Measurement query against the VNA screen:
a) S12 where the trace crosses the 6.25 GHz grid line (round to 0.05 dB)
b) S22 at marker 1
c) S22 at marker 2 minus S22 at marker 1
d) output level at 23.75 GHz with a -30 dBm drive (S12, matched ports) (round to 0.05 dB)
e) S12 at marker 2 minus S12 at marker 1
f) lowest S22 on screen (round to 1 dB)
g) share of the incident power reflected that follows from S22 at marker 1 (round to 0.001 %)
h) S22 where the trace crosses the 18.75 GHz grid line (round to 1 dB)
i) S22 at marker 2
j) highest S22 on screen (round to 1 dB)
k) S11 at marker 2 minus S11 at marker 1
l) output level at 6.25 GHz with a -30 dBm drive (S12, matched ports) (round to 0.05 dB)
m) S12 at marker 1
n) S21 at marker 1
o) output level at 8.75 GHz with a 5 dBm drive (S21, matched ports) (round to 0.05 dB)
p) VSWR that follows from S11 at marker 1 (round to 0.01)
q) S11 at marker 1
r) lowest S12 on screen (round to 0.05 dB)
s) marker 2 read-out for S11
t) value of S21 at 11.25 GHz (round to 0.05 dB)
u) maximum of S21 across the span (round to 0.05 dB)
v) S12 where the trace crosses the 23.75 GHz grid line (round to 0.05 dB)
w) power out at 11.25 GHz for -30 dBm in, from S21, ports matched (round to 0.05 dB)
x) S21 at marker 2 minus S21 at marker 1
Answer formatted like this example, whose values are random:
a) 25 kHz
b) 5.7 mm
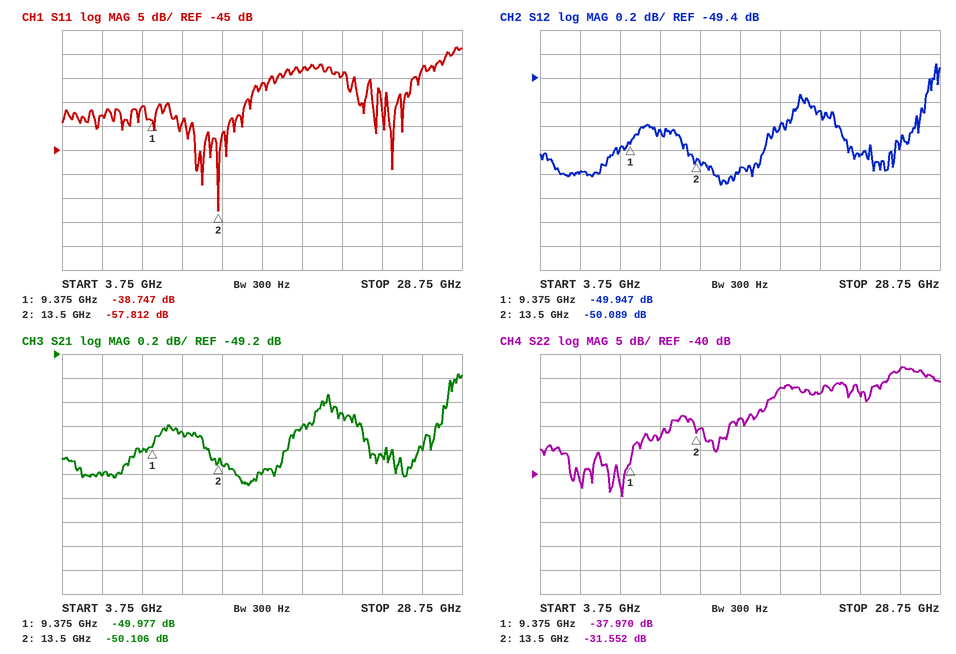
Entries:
a) -50.20 dB
b) -37.970 dB
c) 6.418 dB
d) -80.05 dBm
e) -0.142 dB
f) -45 dB
g) 0.016 %
h) -22 dB
i) -31.552 dB
j) -18 dB
k) -19.065 dB
l) -80.20 dBm
m) -49.947 dB
n) -49.977 dB
o) -45.00 dBm
p) 1.02
q) -38.747 dB
r) -50.30 dB
s) -57.812 dB
t) -49.85 dB
u) -49.35 dB
v) -50.05 dB
w) -79.85 dBm
x) -0.129 dB
